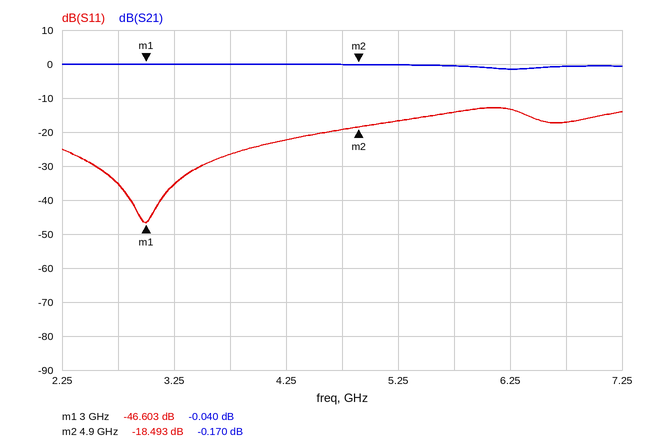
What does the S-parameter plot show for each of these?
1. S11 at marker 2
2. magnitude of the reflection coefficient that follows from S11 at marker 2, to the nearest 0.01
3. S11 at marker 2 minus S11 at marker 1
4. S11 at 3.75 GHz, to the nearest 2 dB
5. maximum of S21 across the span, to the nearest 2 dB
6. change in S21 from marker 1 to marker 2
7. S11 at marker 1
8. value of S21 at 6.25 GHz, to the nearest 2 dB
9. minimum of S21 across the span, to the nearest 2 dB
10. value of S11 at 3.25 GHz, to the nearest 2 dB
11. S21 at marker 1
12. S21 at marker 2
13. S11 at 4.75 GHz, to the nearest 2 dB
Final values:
-18.493 dB
0.12
28.110 dB
-26 dB
0 dB
-0.130 dB
-46.603 dB
-2 dB
-2 dB
-36 dB
-0.040 dB
-0.170 dB
-20 dB
